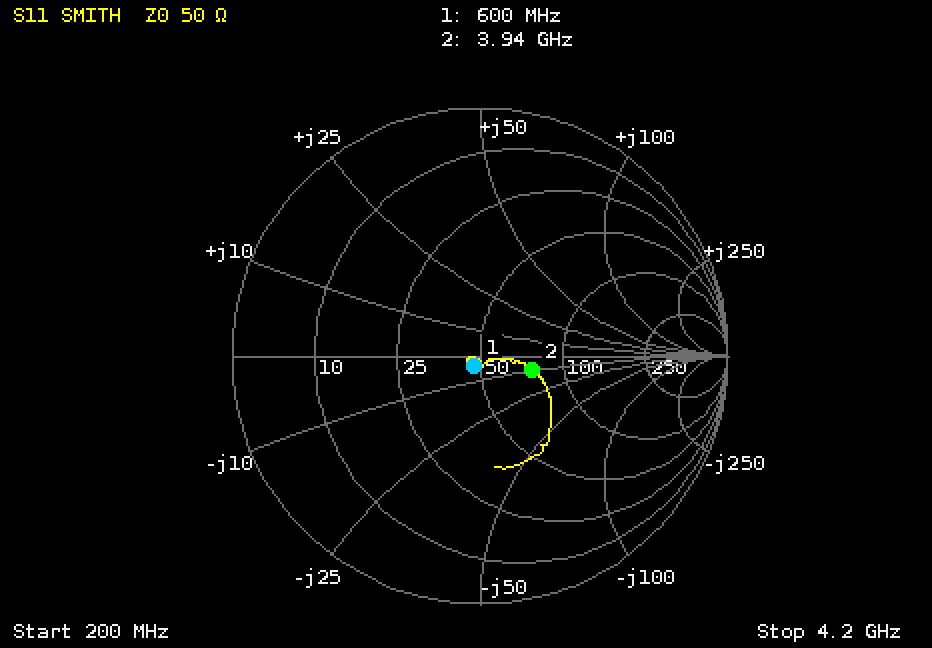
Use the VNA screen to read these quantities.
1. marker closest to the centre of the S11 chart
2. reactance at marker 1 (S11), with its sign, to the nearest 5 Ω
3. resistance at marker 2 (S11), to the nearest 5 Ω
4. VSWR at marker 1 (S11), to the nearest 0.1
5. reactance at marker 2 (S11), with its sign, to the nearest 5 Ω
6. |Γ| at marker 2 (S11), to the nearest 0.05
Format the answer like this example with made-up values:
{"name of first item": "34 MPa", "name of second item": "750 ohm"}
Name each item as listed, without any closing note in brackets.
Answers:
{"marker closest to the centre of the S11 chart": "marker 1", "reactance at marker 1 (S11), with its sign, to the nearest 5 Ω": "-5 Ω", "resistance at marker 2 (S11), to the nearest 5 Ω": "75 Ω", "VSWR at marker 1 (S11), to the nearest 0.1": "1.1", "reactance at marker 2 (S11), with its sign, to the nearest 5 Ω": "-10 Ω", "|Γ| at marker 2 (S11), to the nearest 0.05": "0.20"}
